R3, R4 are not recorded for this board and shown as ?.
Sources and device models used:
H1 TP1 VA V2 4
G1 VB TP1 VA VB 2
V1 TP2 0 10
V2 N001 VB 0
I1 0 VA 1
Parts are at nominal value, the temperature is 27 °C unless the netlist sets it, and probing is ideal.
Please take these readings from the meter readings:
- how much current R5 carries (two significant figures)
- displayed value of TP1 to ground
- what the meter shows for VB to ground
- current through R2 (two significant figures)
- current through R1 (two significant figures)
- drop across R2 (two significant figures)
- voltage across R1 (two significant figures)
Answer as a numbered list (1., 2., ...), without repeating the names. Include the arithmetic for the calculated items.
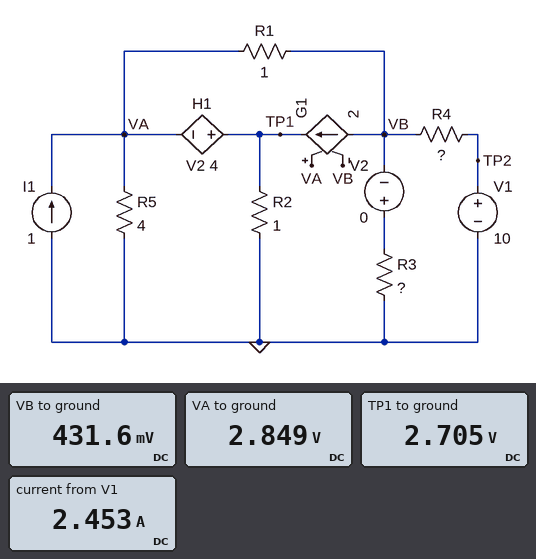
1. (2.849 V) / 4 Ω = 710 mA
2. 2.705 V
3. 431.6 mV
4. (2.705 V) / 1 Ω = 2.7 A
5. (2.849 V - 431.6 mV) / 1 Ω = 2.4 A
6. 2.705 V = 2.7 V
7. 2.849 V - 431.6 mV = 2.4 V
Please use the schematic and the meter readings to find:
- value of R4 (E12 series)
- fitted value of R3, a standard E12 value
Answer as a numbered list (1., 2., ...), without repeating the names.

1. 3.9 Ω
2. 12 Ω
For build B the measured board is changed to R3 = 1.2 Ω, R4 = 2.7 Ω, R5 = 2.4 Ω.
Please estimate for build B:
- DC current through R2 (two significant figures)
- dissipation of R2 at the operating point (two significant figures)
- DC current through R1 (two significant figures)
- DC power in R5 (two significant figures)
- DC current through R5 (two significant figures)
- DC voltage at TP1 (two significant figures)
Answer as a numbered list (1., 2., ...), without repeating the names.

1. 2.9 A
2. 8.5 W
3. 3.4 A
4. 5.6 W
5. 1.5 A
6. 2.9 V
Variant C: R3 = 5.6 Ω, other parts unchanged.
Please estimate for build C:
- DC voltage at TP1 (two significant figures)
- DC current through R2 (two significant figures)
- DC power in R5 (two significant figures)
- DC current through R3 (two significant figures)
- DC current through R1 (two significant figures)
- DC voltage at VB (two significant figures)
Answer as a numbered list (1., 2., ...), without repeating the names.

1. 2.4 V
2. 2.4 A
3. 2.3 W
4. 150 mA
5. 2.2 A
6. 840 mV
